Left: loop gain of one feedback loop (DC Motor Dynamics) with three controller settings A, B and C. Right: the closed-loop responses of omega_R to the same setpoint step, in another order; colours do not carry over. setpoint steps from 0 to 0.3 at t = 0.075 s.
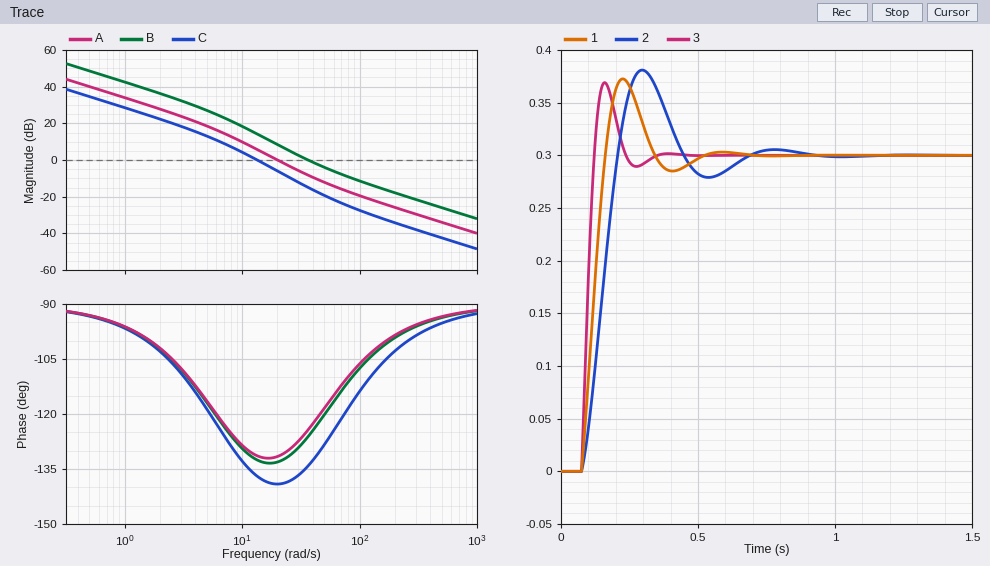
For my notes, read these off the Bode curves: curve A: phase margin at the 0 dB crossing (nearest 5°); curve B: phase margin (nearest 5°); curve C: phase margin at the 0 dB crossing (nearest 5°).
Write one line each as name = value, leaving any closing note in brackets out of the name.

curve A: phase margin at the 0 dB crossing = 50°
curve B: phase margin = 55°
curve C: phase margin at the 0 dB crossing = 45°
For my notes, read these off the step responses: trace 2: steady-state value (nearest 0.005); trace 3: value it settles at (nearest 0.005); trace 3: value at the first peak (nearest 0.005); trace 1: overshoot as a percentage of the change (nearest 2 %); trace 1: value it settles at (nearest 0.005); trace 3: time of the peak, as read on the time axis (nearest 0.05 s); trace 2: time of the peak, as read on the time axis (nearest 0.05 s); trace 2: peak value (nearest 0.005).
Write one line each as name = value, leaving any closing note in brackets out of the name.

trace 2: steady-state value = 0.300
trace 3: value it settles at = 0.300
trace 3: value at the first peak = 0.370
trace 1: overshoot as a percentage of the change = 24 %
trace 1: value it settles at = 0.300
trace 3: time of the peak, as read on the time axis = 0.15 s
trace 2: time of the peak, as read on the time axis = 0.30 s
trace 2: peak value = 0.380
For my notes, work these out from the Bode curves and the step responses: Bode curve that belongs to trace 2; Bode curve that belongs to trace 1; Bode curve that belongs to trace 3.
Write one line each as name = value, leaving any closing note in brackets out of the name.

Bode curve that belongs to trace 2 = C
Bode curve that belongs to trace 1 = A
Bode curve that belongs to trace 3 = B
